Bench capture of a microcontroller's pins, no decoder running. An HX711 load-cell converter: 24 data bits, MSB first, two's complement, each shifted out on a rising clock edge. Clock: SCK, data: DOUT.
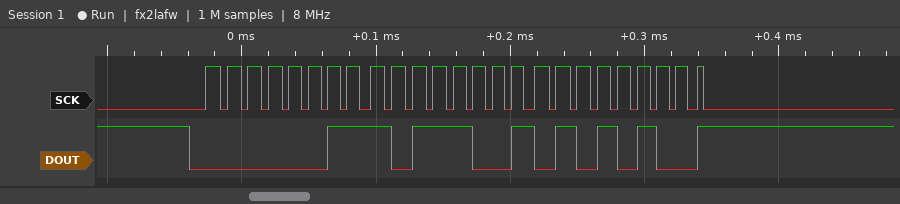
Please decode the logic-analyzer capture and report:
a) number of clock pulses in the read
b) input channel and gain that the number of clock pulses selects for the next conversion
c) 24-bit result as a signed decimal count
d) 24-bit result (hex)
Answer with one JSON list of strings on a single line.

["25", "channel A, gain 128", "244052", "0x03B954"]
